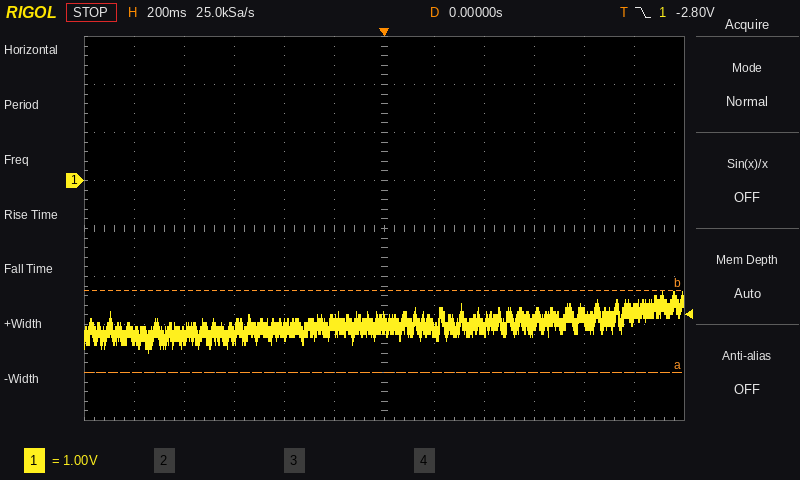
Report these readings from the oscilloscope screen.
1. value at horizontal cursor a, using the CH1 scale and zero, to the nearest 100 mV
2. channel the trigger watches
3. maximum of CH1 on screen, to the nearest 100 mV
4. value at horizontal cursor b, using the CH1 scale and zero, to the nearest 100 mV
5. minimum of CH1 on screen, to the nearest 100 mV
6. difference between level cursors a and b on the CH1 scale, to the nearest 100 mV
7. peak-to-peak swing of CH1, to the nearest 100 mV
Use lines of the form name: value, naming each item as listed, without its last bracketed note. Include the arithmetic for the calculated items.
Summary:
value at horizontal cursor a, using the CH1 scale and zero, to the nearest 100 mV: -4.0 V
channel the trigger watches: CH1
maximum of CH1 on screen, to the nearest 100 mV: -2.3 V
value at horizontal cursor b, using the CH1 scale and zero, to the nearest 100 mV: -2.3 V
minimum of CH1 on screen, to the nearest 100 mV: -3.6 V
difference between level cursors a and b on the CH1 scale, to the nearest 100 mV: 1.7 V
peak-to-peak swing of CH1, to the nearest 100 mV: -2.3 V − (-3.6 V) = 1.3 V
